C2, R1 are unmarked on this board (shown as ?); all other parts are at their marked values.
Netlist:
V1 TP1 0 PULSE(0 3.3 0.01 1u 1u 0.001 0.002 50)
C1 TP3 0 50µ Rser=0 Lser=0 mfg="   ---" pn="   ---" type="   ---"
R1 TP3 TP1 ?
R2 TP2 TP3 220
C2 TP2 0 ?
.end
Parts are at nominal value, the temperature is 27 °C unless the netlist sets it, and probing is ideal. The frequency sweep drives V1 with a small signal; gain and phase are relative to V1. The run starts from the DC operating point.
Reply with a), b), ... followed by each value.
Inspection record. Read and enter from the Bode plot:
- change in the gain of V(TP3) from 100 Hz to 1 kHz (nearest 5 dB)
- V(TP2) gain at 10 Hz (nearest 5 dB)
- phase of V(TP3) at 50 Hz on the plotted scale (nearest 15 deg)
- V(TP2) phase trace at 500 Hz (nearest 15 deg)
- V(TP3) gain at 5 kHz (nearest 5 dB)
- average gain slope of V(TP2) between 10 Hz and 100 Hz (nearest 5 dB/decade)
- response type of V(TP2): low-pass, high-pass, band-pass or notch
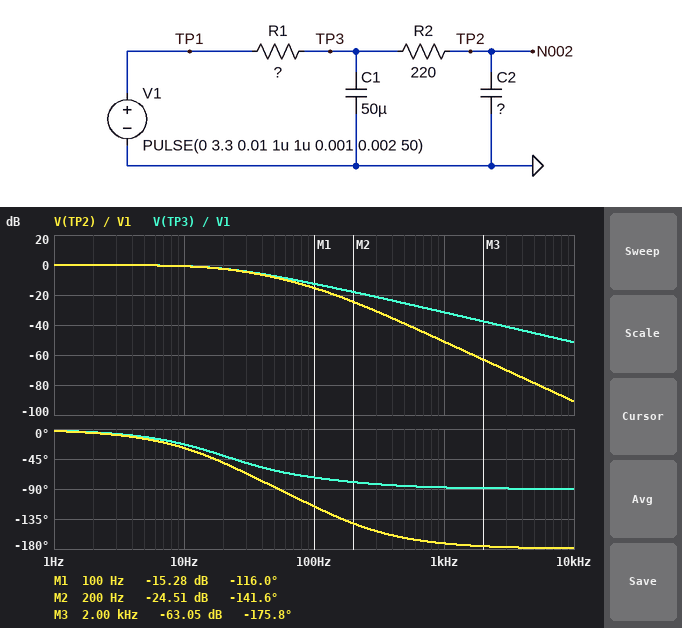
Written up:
a) -20 dB
b) 0 dB
c) -60 deg
d) -165 deg
e) -45 dB
f) -15 dB/decade
g) low-pass
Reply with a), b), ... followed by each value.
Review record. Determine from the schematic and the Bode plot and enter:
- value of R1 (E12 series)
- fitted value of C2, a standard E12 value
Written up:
a) 120 Ω
b) 6.8 µF
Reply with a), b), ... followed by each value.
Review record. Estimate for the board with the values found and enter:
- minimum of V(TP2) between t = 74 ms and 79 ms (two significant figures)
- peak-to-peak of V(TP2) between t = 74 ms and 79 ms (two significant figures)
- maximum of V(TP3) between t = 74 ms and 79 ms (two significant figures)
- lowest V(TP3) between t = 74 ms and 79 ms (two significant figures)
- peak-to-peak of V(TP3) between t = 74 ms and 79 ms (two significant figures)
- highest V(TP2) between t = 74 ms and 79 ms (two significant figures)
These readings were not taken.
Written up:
a) 1.6 V
b) 45 mV
c) 1.8 V
d) 1.5 V
e) 270 mV
f) 1.7 V
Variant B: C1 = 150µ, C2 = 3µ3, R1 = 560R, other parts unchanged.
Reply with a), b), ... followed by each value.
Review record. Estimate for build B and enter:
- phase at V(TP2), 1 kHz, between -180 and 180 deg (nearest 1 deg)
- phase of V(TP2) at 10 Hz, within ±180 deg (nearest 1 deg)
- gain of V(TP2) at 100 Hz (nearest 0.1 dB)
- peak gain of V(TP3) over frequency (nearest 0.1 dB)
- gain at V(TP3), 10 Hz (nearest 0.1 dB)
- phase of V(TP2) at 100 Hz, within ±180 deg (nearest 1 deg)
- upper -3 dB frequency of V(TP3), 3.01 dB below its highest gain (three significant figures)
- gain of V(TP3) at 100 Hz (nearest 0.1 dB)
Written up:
a) -167 deg
b) -82 deg
c) -35.4 dB
d) 0 dB
e) -14.8 dB
f) -113 deg
g) 1.85 Hz
h) -34.6 dB
